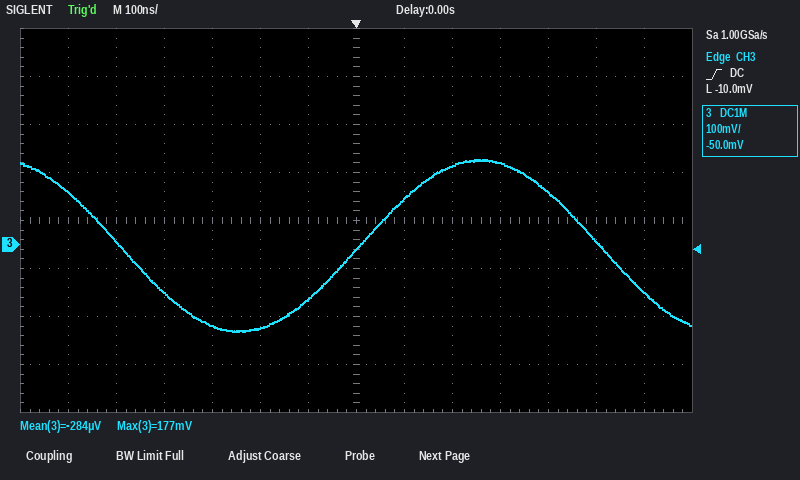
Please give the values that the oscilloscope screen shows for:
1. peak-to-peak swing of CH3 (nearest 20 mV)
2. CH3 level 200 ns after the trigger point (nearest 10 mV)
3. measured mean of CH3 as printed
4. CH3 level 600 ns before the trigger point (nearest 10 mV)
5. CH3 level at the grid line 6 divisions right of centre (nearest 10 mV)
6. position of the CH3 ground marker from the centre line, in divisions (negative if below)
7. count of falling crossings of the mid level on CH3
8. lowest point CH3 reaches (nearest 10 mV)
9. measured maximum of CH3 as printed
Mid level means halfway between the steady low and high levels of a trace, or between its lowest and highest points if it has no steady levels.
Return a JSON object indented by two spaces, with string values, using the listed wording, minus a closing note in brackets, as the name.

{
  "peak-to-peak swing of CH3": "360 mV",
  "CH3 level 200 ns after the trigger point": "160 mV",
  "measured mean of CH3 as printed": "-284 µV",
  "CH3 level 600 ns before the trigger point": "110 mV",
  "CH3 level at the grid line 6 divisions right of centre": "-100 mV",
  "position of the CH3 ground marker from the centre line, in divisions": "-0.5 div",
  "count of falling crossings of the mid level on CH3": "2",
  "lowest point CH3 reaches": "-180 mV",
  "measured maximum of CH3 as printed": "177 mV"
}
